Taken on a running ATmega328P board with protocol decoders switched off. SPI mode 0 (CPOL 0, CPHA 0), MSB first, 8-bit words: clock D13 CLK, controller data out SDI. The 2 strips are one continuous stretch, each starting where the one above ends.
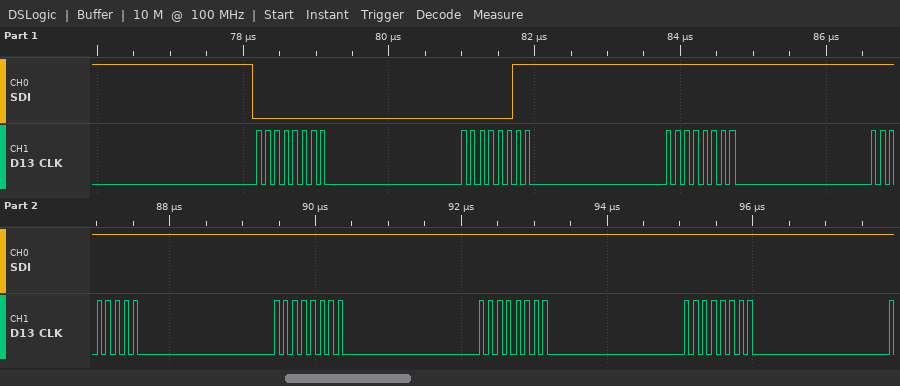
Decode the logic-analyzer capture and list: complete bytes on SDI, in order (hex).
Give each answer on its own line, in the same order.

00 03 FF FF FF FF FF
